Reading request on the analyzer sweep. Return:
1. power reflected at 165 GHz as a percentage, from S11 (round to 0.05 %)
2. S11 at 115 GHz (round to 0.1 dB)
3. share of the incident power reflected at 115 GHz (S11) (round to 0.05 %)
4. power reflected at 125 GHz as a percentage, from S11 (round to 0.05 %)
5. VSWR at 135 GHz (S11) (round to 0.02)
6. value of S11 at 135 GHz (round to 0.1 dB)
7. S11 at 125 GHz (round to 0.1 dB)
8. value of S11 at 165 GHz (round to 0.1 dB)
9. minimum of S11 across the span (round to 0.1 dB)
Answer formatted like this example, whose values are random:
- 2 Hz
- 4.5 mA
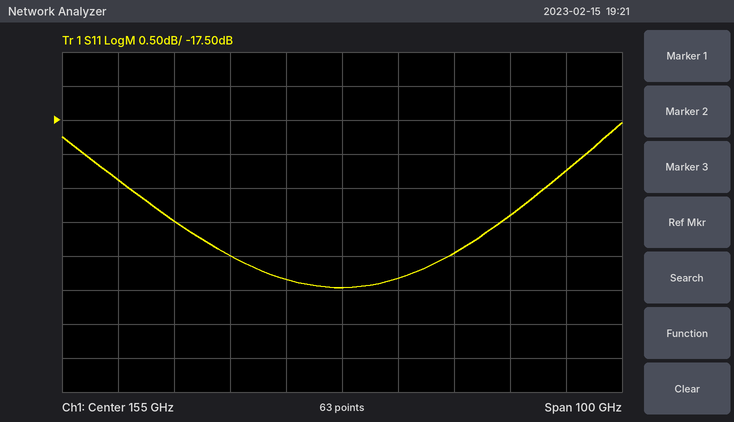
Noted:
- 1.05 %
- -18.4 dB
- 1.45 %
- 1.25 %
- 1.24
- -19.5 dB
- -19.0 dB
- -19.8 dB
- -20.0 dB
